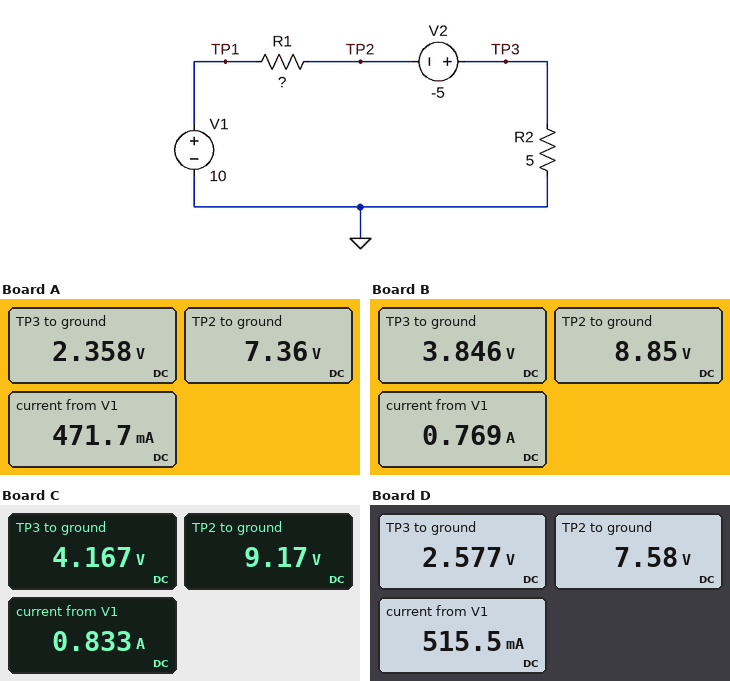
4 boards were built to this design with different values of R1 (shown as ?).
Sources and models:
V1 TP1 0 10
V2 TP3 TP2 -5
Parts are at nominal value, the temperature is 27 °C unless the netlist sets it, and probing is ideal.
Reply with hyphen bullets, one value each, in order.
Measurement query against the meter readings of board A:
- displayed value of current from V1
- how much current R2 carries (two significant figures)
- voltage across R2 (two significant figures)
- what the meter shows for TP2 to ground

- 471.7 mA
- 470 mA
- 2.4 V
- 7.36 V
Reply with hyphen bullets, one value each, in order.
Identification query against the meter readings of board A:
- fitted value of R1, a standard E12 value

- 5.6 Ω
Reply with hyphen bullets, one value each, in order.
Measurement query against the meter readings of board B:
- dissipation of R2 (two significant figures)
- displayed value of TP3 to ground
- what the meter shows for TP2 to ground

- 3.0 W
- 3.846 V
- 8.85 V
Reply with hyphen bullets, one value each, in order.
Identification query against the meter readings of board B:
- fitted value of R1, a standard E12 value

- 1.5 Ω
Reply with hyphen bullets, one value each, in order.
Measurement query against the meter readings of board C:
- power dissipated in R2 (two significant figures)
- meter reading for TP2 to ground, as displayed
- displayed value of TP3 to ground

- 3.5 W
- 9.17 V
- 4.167 V
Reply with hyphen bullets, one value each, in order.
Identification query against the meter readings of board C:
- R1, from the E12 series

- 1 Ω
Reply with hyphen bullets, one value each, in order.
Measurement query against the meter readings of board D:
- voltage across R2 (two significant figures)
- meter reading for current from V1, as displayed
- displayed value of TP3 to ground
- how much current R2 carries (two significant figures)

- 2.6 V
- 515.5 mA
- 2.577 V
- 520 mA
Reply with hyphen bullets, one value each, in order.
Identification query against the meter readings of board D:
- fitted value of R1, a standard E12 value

- 4.7 Ω
